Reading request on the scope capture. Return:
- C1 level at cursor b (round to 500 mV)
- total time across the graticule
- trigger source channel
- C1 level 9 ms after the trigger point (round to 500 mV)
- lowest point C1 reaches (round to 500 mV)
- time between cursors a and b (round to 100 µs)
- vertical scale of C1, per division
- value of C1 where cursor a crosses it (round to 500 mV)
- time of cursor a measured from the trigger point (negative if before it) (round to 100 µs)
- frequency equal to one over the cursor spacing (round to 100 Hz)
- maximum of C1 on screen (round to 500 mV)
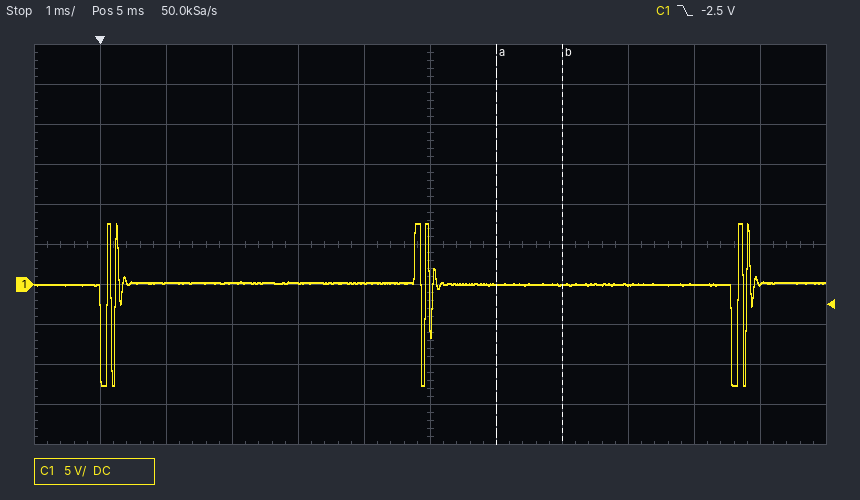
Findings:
0.0 V
12 ms
C1
0.0 V
-12.5 V
1.0 ms
5 V
0.0 V
+6.0 ms
1.0 kHz
7.5 V
